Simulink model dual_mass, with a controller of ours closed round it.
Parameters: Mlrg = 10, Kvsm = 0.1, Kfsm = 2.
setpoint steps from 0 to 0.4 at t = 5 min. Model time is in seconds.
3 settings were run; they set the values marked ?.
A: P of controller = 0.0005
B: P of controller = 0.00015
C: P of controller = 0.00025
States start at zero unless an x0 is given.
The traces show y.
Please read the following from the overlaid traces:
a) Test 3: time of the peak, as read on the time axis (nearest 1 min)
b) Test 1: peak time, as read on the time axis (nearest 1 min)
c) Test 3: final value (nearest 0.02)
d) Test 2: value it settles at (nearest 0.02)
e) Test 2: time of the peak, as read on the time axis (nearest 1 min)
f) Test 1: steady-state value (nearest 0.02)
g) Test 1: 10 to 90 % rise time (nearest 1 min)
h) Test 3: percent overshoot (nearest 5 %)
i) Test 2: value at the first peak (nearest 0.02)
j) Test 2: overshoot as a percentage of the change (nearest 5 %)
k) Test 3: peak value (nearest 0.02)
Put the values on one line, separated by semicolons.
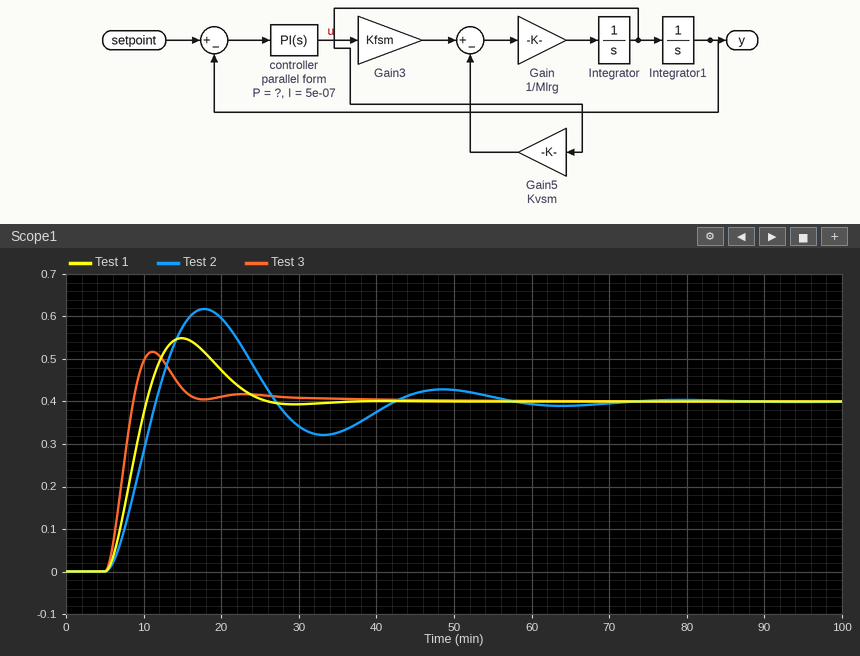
11 min; 15 min; 0.40; 0.40; 18 min; 0.40; 4 min; 30 %; 0.62; 55 %; 0.52
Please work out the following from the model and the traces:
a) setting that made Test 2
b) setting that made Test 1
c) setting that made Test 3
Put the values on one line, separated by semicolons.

B; C; A
